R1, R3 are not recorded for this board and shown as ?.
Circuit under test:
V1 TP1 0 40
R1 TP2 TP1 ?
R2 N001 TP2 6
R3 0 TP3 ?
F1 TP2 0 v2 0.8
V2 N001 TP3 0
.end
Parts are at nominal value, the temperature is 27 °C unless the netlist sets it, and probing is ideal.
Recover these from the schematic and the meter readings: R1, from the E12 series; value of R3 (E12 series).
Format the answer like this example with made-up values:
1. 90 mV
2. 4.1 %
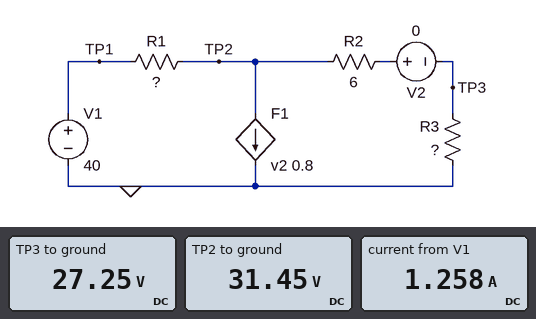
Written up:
1. 6.8 Ω
2. 39 Ω
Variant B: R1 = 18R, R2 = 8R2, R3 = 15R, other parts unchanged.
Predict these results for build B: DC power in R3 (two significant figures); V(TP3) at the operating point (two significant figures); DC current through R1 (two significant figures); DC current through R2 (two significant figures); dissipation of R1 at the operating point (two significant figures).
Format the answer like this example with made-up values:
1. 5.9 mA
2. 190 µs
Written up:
1. 7.8 W
2. 11 V
3. 1.3 A
4. 720 mA
5. 30 W
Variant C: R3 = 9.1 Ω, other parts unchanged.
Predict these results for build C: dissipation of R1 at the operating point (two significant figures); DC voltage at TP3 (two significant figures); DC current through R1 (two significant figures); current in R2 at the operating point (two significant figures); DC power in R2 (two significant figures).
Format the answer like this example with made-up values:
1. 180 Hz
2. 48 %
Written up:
1. 47 W
2. 13 V
3. 2.6 A
4. 1.5 A
5. 13 W
